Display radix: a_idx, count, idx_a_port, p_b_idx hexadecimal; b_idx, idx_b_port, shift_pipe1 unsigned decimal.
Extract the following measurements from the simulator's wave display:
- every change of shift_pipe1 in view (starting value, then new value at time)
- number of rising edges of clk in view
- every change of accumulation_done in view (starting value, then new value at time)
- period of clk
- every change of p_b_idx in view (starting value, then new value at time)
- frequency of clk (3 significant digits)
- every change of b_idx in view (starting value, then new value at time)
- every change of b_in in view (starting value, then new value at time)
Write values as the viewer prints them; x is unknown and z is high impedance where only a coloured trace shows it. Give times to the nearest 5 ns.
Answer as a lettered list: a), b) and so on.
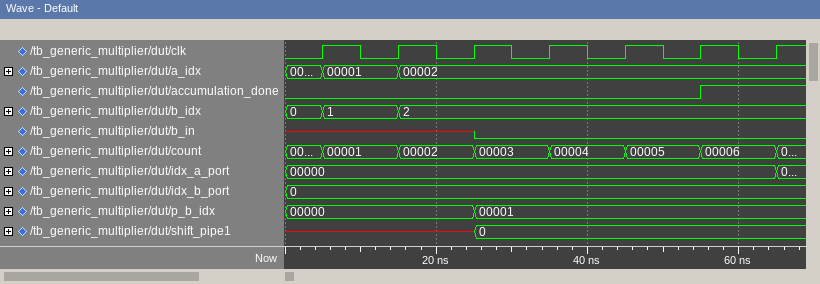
a) x, 0 at 25 ns
b) 7
c) 0, 1 at 55 ns
d) 10 ns
e) 00000, 00001 at 25 ns
f) 100 MHz
g) 0, 1 at 5 ns, 2 at 15 ns
h) x, 0 at 25 ns
